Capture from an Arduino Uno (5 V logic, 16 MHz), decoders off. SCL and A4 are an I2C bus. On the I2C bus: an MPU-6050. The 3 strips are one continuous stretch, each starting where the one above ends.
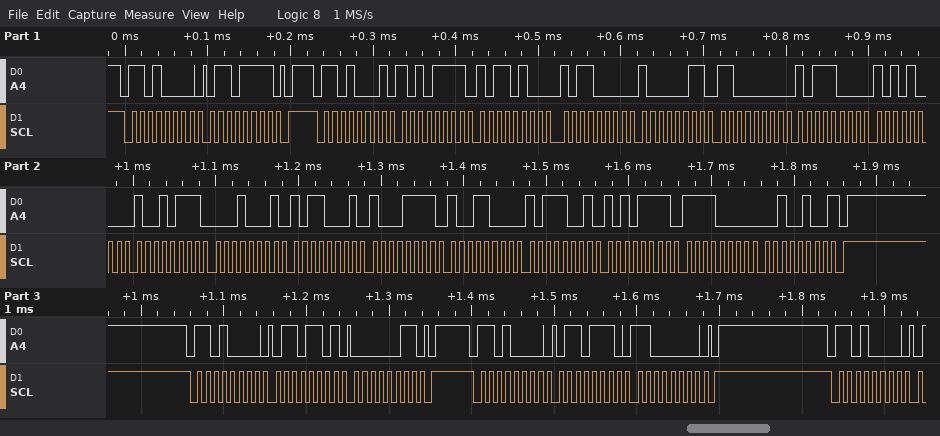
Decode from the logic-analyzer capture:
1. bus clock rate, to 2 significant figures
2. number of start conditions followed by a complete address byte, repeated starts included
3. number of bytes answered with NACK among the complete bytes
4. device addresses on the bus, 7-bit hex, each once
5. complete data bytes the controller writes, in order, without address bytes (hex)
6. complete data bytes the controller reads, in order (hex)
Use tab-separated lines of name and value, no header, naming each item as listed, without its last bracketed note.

bus clock rate, to 2 significant figures	100 kHz
number of start conditions followed by a complete address byte, repeated starts included	5
number of bytes answered with NACK among the complete bytes	1
device addresses on the bus, 7-bit hex, each once	0x68
complete data bytes the controller writes, in order, without address bytes	6F 6D 03 6E C0
complete data bytes the controller reads, in order	AF B4 B0 83 C0 B8 A8 97 11 B1 8F 98 B9 AF F0 24
